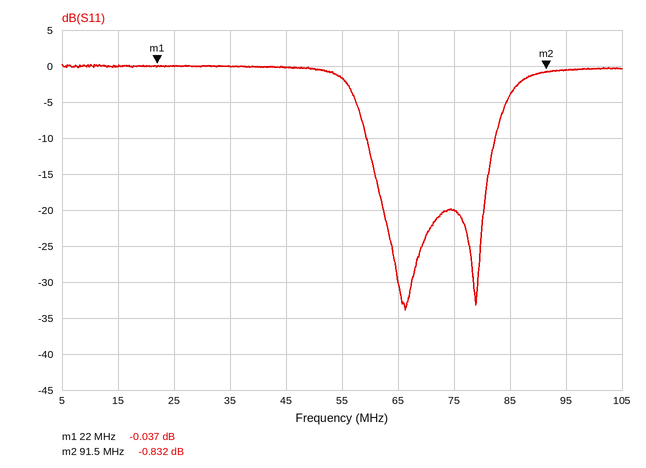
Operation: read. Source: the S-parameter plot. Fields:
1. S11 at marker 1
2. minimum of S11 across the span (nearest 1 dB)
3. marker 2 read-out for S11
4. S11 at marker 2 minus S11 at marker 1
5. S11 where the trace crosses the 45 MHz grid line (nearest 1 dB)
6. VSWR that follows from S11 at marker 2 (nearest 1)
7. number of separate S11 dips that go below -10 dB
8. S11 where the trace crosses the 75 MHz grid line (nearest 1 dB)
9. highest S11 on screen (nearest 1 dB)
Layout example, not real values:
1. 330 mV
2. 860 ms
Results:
1. -0.037 dB
2. -34 dB
3. -0.832 dB
4. -0.795 dB
5. 0 dB
6. 21
7. 2
8. -20 dB
9. 0 dB
